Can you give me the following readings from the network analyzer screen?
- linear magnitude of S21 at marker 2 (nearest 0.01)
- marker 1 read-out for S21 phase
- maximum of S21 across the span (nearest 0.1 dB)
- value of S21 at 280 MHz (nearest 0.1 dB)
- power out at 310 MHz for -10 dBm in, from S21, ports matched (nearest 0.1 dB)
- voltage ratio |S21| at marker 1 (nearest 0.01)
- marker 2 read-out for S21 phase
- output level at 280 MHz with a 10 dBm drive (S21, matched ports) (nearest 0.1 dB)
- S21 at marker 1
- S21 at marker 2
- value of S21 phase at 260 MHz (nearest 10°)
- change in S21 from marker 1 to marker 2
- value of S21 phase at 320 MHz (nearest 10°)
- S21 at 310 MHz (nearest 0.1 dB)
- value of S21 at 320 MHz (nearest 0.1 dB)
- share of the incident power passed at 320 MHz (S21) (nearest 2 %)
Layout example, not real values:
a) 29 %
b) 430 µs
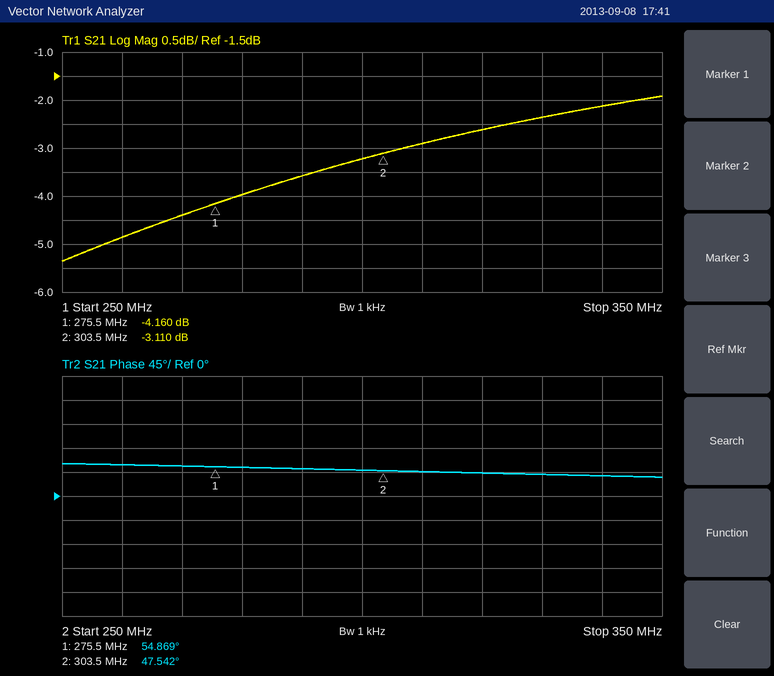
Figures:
a) 0.70
b) 54.869°
c) -1.9 dB
d) -4.0 dB
e) -12.9 dBm
f) 0.62
g) 47.542°
h) 6.0 dBm
i) -4.160 dB
j) -3.110 dB
k) 60°
l) 1.050 dB
m) 40°
n) -2.9 dB
o) -2.6 dB
p) 54 %
